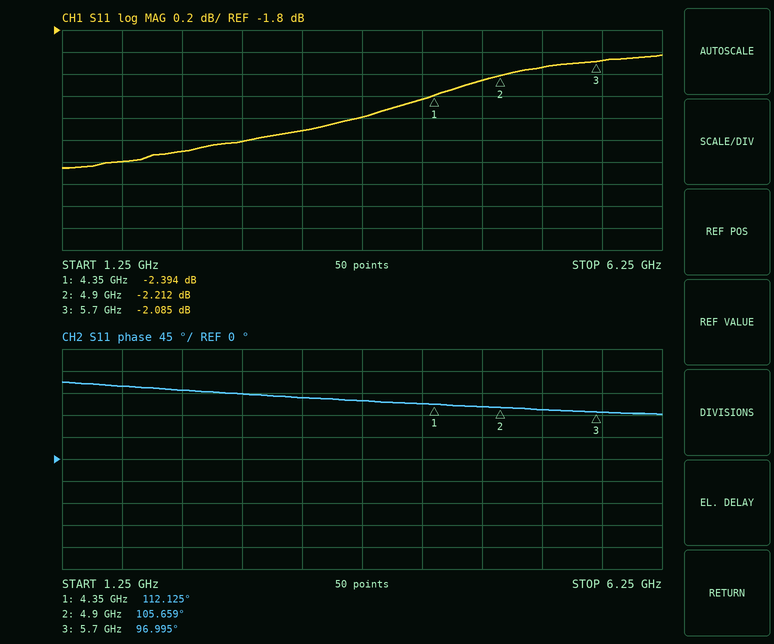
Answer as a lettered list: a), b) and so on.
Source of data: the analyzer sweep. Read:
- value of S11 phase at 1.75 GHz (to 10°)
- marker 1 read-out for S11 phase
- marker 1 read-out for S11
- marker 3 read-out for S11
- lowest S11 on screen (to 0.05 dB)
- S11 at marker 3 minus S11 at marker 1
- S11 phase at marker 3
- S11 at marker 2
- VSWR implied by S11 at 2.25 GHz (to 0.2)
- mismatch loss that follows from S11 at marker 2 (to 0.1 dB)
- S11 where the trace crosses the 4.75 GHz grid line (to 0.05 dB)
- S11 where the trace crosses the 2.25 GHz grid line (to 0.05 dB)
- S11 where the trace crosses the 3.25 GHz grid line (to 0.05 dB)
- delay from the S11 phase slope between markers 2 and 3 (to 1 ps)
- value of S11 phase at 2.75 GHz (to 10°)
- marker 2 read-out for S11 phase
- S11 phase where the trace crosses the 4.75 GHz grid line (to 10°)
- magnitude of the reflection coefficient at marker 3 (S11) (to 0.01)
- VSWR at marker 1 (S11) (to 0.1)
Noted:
a) 150°
b) 112.125°
c) -2.394 dB
d) -2.085 dB
e) -3.05 dB
f) 0.309 dB
g) 96.995°
h) -2.212 dB
i) 6.0
j) 4.0 dB
k) -2.25 dB
l) -2.90 dB
m) -2.70 dB
n) 30 ps
o) 130°
p) 105.659°
q) 110°
r) 0.79
s) 7.3
